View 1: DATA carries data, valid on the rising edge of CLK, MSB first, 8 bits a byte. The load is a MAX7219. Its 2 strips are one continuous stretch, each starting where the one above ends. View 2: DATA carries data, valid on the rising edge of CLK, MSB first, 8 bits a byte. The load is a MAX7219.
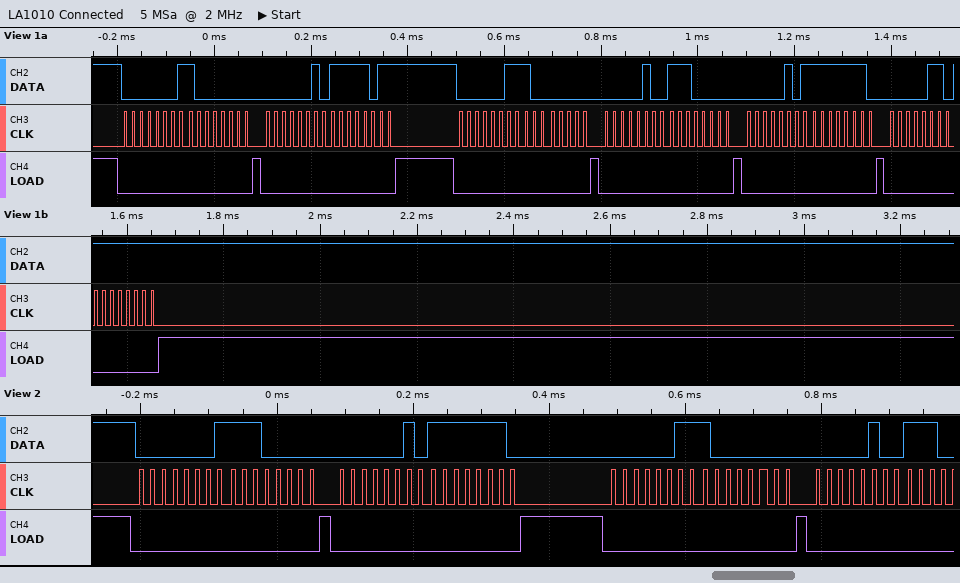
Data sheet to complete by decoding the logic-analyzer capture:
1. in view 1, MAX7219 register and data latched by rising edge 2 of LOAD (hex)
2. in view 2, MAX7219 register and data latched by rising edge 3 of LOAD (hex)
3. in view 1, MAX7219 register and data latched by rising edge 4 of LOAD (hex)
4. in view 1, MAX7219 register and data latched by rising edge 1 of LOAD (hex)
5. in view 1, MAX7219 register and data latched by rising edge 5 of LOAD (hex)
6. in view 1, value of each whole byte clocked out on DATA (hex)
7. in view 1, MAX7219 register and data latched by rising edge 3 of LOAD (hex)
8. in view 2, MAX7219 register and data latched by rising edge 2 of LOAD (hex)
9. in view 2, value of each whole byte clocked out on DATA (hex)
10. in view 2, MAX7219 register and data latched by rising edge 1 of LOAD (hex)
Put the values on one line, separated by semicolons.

register 0x2, data 0xFB; register 0x3, data 0x80; register 0x4, data 0xE0; register 0x1, data 0x80; register 0x5, data 0xFE; 01 80 02 FB 03 80 04 E0 05 FE 06 FF; register 0x3, data 0x80; register 0x2, data 0xFE; 01 E0 02 FE 03 80 04; register 0x1, data 0xE0
